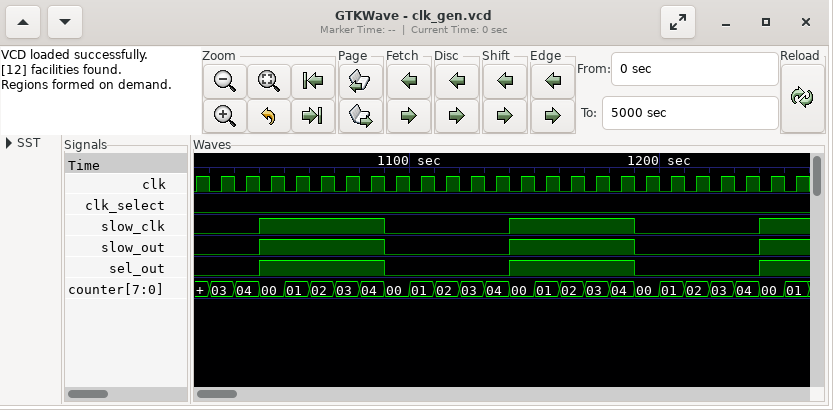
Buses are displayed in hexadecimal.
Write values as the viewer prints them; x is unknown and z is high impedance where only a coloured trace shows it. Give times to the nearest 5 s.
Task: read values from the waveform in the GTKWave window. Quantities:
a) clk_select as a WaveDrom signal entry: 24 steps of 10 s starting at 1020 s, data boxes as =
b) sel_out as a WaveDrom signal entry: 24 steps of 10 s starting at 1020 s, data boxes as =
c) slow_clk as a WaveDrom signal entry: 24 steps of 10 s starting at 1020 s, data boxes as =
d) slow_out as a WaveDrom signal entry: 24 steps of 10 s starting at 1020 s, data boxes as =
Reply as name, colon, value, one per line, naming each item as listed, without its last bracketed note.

clk_select as a WaveDrom signal entry: 24 steps of 10 s starting at 1020 s, data boxes as =: {name: 'clk_select', wave: '0.......................'}
sel_out as a WaveDrom signal entry: 24 steps of 10 s starting at 1020 s, data boxes as =: {name: 'sel_out', wave: '0.1....0....1....0....1.'}
slow_clk as a WaveDrom signal entry: 24 steps of 10 s starting at 1020 s, data boxes as =: {name: 'slow_clk', wave: '0.1....0....1....0....1.'}
slow_out as a WaveDrom signal entry: 24 steps of 10 s starting at 1020 s, data boxes as =: {name: 'slow_out', wave: '0.1....0....1....0....1.'}
